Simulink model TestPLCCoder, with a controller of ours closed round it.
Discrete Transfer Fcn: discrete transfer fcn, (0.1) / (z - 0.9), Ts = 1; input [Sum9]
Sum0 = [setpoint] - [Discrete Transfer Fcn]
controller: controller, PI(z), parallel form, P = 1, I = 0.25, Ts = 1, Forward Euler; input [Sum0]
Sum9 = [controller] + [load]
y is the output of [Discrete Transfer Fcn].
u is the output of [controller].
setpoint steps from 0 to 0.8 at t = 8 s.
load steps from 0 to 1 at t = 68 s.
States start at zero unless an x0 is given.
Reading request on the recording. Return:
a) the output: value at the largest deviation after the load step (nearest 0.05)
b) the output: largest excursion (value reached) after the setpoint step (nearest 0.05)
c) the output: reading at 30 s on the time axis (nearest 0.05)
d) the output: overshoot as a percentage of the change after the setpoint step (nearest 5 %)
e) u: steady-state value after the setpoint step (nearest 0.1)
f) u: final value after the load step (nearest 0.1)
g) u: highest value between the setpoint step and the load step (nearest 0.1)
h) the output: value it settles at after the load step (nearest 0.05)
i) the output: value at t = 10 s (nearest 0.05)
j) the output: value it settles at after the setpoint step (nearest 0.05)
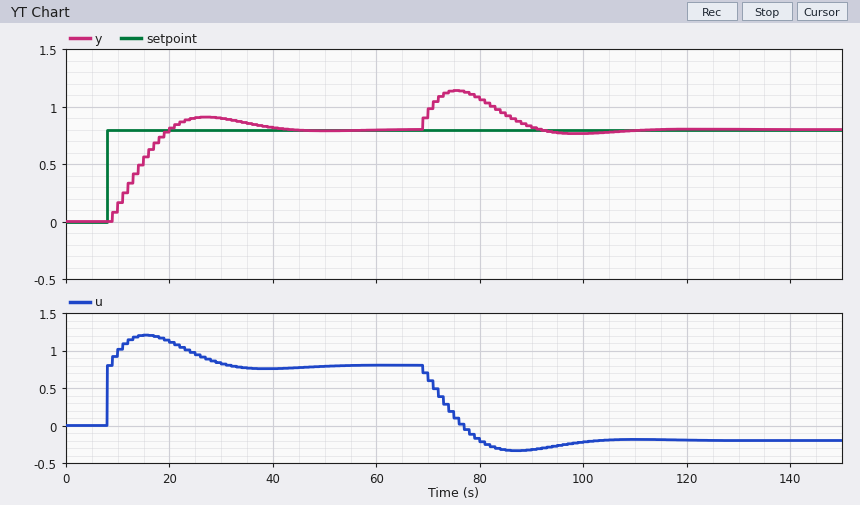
1.15
0.90
0.90
15 %
0.8
-0.2
1.2
0.80
0.15
0.80
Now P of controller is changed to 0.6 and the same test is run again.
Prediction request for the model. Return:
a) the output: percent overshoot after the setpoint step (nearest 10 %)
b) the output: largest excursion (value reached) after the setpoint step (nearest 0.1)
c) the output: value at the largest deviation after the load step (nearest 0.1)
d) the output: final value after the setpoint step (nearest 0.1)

20 %
1.0
1.2
0.8
